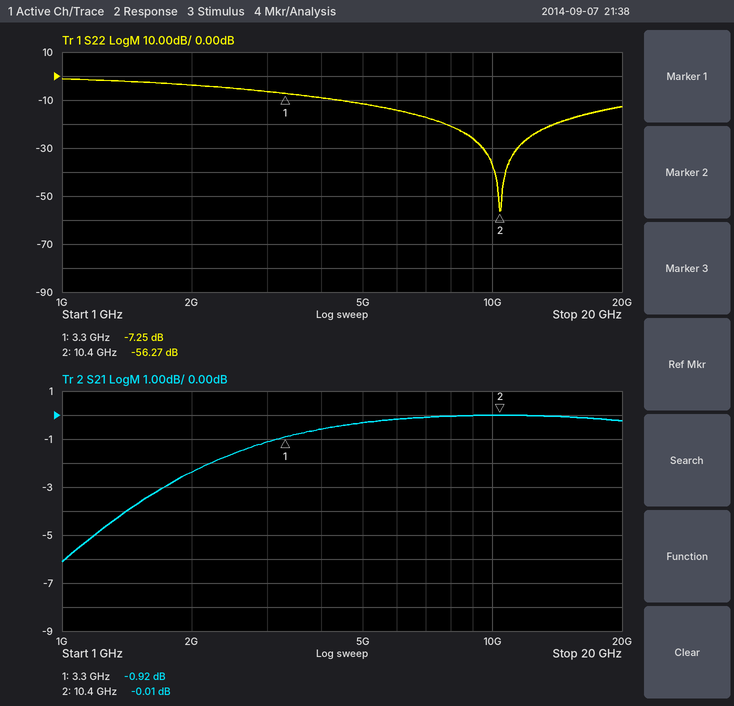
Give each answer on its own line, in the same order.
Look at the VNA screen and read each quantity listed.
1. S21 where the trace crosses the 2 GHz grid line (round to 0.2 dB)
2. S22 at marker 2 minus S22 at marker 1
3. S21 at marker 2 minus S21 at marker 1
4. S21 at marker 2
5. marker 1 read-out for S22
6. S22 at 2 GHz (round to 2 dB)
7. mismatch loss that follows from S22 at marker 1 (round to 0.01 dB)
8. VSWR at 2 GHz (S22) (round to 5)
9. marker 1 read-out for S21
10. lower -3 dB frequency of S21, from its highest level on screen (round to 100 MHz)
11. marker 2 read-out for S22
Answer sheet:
-2.4 dB
-49.02 dB
0.91 dB
-0.01 dB
-7.25 dB
-4 dB
0.91 dB
5
-0.92 dB
1.7 GHz
-56.27 dB
